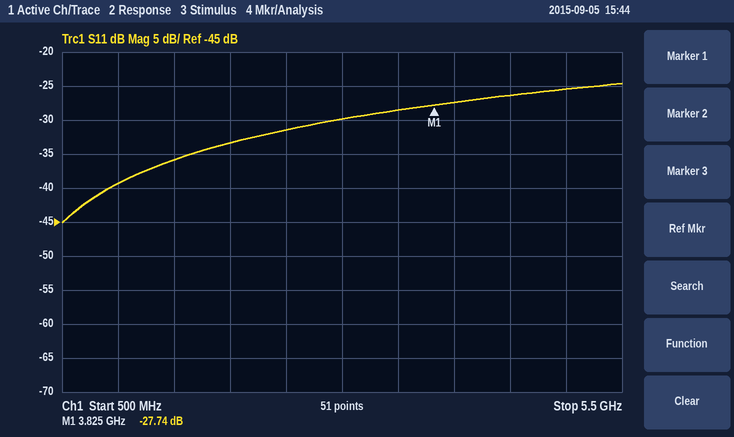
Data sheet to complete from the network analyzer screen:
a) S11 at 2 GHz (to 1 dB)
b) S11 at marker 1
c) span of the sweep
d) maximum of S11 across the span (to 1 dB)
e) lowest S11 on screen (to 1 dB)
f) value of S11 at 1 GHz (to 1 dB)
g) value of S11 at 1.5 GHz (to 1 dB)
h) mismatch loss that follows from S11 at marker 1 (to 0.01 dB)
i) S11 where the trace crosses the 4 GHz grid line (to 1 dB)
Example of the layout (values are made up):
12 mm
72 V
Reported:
-33 dB
-27.74 dB
5 GHz
-25 dB
-45 dB
-39 dB
-36 dB
0.01 dB
-27 dB
